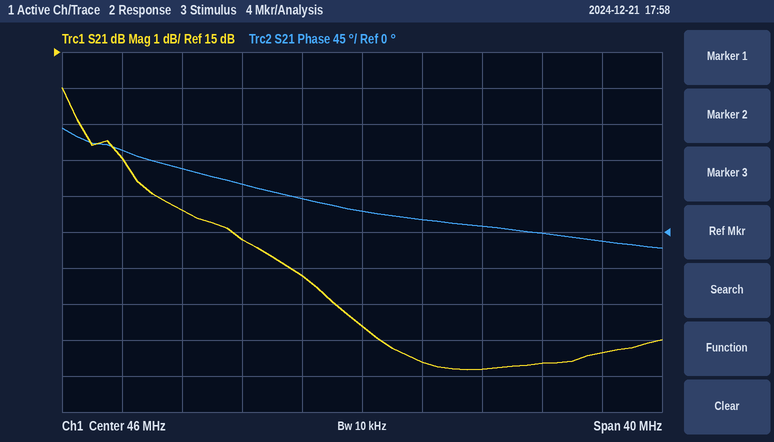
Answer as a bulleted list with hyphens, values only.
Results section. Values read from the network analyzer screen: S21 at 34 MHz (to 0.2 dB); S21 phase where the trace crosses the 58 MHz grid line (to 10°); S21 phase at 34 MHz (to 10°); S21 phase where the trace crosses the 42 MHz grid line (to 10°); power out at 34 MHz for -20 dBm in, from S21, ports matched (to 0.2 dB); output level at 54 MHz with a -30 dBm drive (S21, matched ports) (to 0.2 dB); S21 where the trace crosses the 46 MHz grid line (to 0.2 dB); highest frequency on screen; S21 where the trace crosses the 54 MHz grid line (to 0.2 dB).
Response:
- 10.6 dB
- 0°
- 80°
- 40°
- -9.4 dBm
- -23.8 dBm
- 7.4 dB
- 66 MHz
- 6.2 dB
